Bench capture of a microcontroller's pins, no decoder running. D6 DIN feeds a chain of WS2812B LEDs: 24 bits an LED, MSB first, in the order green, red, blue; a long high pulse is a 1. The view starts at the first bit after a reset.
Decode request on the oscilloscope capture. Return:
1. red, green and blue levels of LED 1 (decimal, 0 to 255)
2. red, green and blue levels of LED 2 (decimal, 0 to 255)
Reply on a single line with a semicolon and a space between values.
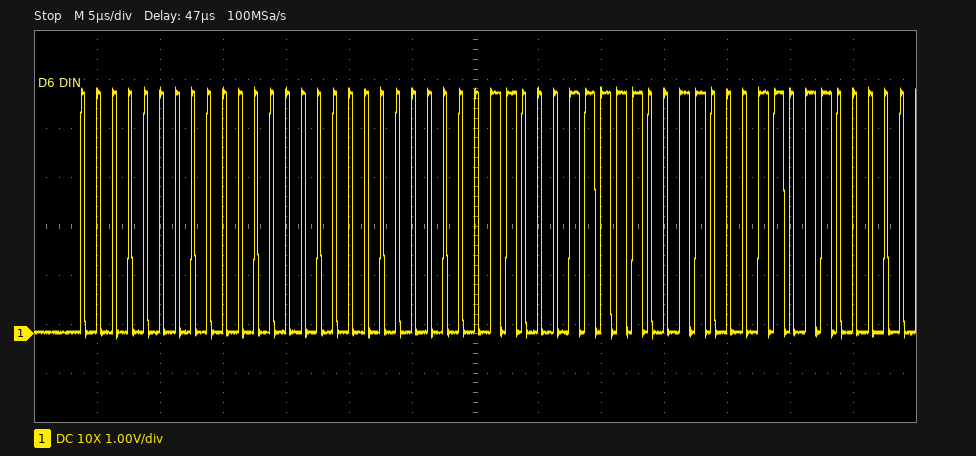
0, 0, 0; 243, 49, 27
